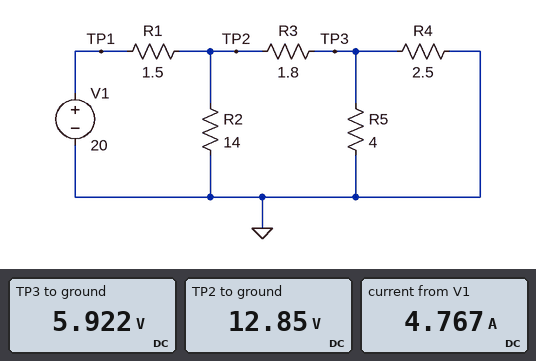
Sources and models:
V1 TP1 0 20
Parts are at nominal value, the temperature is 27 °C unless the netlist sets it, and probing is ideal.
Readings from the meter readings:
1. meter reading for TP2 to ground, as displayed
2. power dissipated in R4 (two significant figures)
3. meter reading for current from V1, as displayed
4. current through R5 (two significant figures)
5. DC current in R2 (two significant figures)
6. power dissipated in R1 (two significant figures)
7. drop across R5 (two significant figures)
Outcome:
12.85 V
14 W
4.767 A
1.5 A
920 mA
34 W
5.9 V
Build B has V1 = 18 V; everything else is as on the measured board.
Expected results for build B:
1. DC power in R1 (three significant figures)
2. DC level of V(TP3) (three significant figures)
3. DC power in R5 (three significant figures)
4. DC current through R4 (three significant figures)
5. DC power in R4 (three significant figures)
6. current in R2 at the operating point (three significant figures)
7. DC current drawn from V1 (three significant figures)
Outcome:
27.6 W
5.33 V
7.10 W
2.13 A
11.4 W
826 mA
4.29 A
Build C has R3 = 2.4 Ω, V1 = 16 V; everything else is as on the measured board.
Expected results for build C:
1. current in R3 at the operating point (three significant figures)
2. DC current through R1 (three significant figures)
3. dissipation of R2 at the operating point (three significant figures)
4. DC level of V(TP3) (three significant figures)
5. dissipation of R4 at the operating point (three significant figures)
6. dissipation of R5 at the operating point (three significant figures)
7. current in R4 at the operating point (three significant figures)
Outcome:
2.73 A
3.50 A
8.26 W
4.20 V
7.06 W
4.41 W
1.68 A
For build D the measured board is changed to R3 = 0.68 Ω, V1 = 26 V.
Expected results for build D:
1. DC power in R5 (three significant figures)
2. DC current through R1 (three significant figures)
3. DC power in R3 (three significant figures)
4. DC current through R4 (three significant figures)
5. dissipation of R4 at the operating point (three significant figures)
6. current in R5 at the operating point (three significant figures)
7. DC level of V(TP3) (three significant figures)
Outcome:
25.6 W
7.61 A
29.4 W
4.04 A
40.9 W
2.53 A
10.1 V
